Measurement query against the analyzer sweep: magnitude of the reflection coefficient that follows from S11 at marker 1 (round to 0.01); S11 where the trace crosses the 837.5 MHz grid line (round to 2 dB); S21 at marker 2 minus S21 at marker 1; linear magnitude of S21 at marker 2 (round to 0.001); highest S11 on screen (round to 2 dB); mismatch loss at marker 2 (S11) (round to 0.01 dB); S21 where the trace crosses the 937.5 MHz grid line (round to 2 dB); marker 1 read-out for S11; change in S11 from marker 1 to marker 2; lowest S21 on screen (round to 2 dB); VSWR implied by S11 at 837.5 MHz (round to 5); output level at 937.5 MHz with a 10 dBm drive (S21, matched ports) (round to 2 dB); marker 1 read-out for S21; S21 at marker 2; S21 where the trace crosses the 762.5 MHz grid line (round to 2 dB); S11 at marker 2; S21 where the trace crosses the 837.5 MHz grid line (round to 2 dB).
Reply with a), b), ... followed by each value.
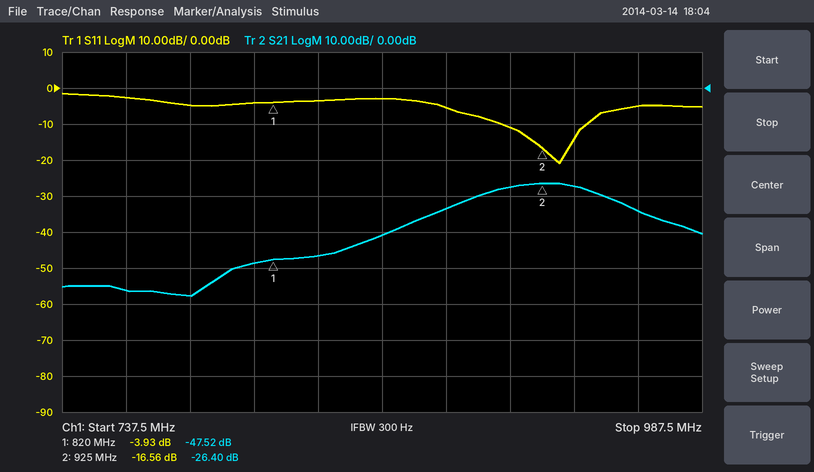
a) 0.64
b) -4 dB
c) 21.12 dB
d) 0.048
e) -2 dB
f) 0.10 dB
g) -28 dB
h) -3.93 dB
i) -12.63 dB
j) -58 dB
k) 5
l) -18 dBm
m) -47.52 dB
n) -26.40 dB
o) -56 dB
p) -16.56 dB
q) -46 dB
